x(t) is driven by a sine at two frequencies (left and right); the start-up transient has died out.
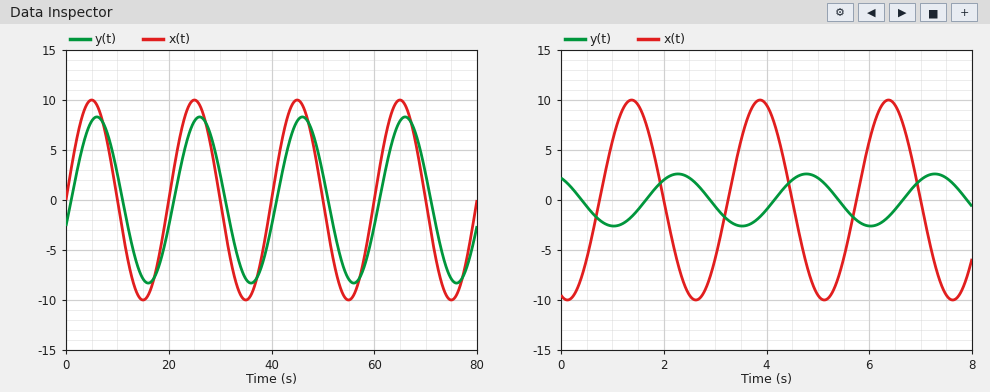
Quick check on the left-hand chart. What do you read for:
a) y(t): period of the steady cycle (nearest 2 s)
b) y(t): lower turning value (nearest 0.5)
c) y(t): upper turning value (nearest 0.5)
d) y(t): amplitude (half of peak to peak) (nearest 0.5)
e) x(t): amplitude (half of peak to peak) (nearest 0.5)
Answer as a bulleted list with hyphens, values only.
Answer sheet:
- 20 s
- -8.5
- 8.5
- 8.5
- 10.0
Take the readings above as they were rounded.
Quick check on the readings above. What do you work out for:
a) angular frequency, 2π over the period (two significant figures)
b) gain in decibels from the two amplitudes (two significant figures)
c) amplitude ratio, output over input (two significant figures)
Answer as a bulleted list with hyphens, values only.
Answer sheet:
- 0.31 rad/s
- -1.4 dB
- 0.85
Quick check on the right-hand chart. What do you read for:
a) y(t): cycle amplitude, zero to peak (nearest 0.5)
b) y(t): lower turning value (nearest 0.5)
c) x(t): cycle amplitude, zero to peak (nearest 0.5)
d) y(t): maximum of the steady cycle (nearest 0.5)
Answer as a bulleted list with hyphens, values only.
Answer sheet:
- 2.5
- -2.5
- 10.0
- 2.5
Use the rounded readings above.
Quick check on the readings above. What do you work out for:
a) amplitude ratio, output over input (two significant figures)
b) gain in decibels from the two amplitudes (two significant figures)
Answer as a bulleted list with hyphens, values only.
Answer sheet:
- 0.25
- -12 dB
